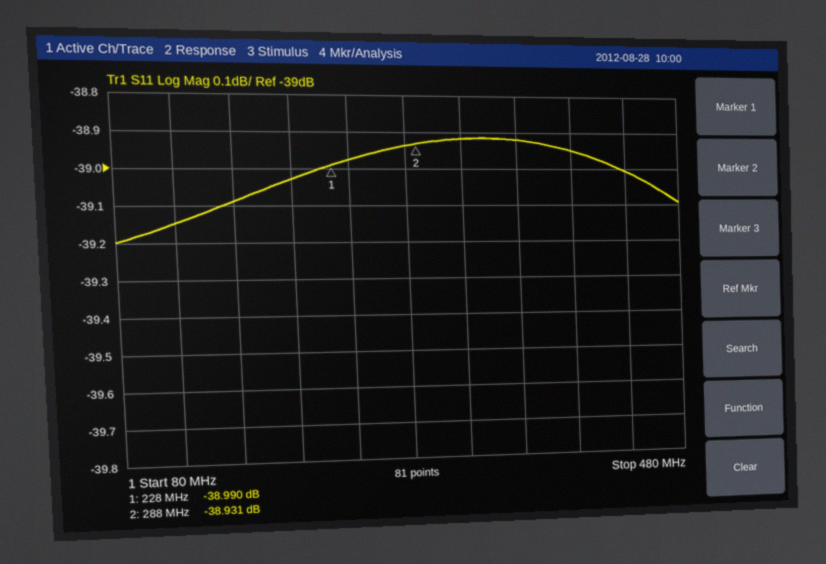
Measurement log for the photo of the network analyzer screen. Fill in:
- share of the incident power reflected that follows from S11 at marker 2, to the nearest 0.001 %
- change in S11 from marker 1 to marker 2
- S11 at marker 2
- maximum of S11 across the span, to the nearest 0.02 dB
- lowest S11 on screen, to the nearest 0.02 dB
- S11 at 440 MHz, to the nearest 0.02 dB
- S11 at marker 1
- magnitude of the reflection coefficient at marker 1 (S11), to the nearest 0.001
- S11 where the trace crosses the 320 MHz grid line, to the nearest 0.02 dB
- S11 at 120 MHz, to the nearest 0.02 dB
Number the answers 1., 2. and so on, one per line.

1. 0.013 %
2. 0.059 dB
3. -38.931 dB
4. -38.92 dB
5. -39.20 dB
6. -39.00 dB
7. -38.990 dB
8. 0.011
9. -38.92 dB
10. -39.14 dB
